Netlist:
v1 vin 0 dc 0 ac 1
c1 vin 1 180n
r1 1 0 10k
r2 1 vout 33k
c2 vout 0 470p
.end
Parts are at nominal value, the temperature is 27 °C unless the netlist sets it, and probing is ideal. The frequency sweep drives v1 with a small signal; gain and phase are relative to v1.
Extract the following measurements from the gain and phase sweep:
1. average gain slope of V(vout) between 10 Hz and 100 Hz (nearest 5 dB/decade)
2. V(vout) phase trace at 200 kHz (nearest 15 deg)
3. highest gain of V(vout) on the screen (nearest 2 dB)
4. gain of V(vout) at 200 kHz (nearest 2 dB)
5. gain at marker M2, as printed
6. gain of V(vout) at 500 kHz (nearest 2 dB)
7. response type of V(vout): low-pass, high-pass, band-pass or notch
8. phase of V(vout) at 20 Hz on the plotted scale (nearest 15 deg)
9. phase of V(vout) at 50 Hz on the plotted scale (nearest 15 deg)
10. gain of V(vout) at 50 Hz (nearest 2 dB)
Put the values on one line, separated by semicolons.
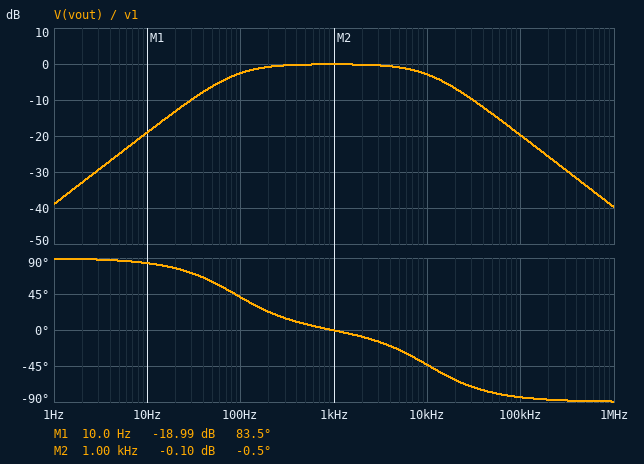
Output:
15 dB/decade; -90 deg; 0 dB; -26 dB; -0.10 dB; -34 dB; band-pass; 75 deg; 60 deg; -6 dB
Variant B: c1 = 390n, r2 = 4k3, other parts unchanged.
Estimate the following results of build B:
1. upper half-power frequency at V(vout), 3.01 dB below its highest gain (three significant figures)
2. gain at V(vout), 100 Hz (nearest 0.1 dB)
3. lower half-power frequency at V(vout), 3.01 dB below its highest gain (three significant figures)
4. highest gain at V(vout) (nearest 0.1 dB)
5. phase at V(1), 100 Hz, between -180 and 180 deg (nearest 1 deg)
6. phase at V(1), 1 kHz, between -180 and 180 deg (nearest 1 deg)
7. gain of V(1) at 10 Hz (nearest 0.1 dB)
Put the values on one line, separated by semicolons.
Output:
78.9 kHz; -0.7 dB; 40.7 Hz; 0 dB; 22 deg; 2 deg; -12.5 dB
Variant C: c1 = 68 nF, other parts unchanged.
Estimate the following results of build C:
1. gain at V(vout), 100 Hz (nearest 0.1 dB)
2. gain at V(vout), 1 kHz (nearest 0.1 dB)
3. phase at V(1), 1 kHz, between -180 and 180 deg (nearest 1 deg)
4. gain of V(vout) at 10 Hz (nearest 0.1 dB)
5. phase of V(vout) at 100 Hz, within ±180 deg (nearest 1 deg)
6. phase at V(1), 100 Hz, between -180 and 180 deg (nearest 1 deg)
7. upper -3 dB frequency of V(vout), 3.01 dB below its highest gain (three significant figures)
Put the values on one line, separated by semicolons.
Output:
-8.1 dB; -0.3 dB; 13 deg; -27.4 dB; 66 deg; 67 deg; 10.8 kHz
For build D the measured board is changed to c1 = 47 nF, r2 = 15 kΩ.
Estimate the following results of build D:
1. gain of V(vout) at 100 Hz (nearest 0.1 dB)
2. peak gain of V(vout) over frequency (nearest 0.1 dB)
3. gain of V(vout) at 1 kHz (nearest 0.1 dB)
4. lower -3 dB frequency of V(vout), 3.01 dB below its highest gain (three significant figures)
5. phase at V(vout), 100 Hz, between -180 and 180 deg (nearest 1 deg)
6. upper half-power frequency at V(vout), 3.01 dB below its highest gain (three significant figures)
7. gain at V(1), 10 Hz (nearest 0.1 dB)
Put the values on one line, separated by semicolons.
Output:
-11.0 dB; -0.2 dB; -0.6 dB; 326 Hz; 73 deg; 23.5 kHz; -30.6 dB
